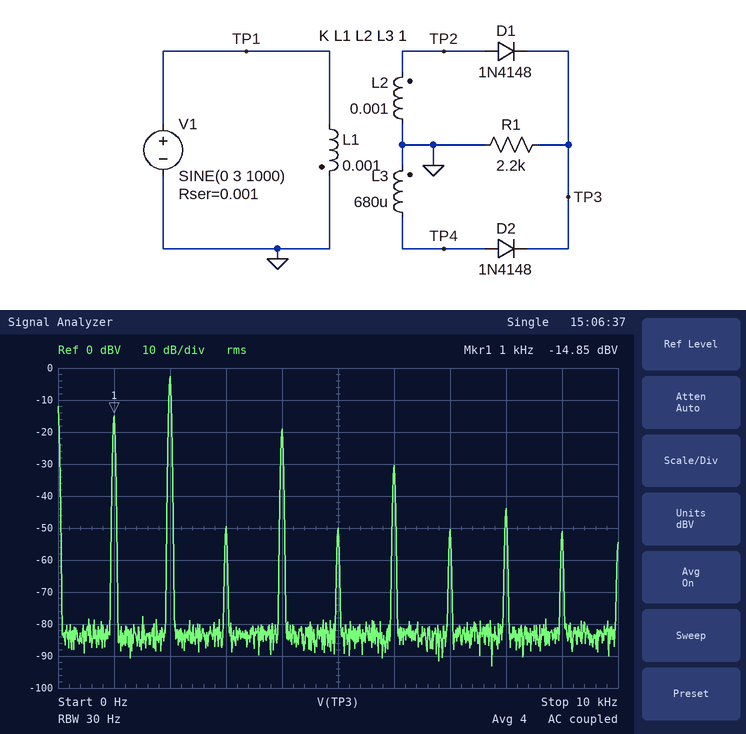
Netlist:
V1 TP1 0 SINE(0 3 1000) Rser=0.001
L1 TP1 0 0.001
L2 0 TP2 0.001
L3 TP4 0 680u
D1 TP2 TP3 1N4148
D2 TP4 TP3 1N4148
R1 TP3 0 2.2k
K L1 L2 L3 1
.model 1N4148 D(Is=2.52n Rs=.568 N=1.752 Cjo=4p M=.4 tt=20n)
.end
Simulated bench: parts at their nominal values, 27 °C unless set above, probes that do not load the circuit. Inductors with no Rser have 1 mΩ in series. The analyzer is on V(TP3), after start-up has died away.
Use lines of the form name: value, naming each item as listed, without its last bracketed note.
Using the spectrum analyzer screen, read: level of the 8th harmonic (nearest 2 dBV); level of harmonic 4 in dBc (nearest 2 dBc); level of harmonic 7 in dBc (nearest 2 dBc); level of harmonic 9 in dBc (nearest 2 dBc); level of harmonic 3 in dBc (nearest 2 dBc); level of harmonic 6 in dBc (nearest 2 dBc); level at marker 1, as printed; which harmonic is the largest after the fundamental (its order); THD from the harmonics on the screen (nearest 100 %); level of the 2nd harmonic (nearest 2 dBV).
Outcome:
level of the 8th harmonic: -44 dBV
level of harmonic 4 in dBc: -4 dBc
level of harmonic 7 in dBc: -36 dBc
level of harmonic 9 in dBc: -36 dBc
level of harmonic 3 in dBc: -34 dBc
level of harmonic 6 in dBc: -16 dBc
level at marker 1, as printed: -14.85 dBV
which harmonic is the largest after the fundamental: 2
THD from the harmonics on the screen: 400 %
level of the 2nd harmonic: -2 dBV
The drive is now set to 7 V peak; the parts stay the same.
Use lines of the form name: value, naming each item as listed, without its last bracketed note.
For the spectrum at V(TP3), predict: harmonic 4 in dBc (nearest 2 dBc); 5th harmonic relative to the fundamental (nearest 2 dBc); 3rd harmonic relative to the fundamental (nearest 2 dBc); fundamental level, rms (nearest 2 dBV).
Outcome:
harmonic 4 in dBc: -2 dBc
5th harmonic relative to the fundamental: -50 dBc
3rd harmonic relative to the fundamental: -48 dBc
fundamental level, rms: -8 dBV
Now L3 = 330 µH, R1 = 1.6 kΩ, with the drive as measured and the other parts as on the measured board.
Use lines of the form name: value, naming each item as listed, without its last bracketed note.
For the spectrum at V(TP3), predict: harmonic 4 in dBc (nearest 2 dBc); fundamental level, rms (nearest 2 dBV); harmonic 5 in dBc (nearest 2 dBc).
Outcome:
harmonic 4 in dBc: -14 dBc
fundamental level, rms: -8 dBV
harmonic 5 in dBc: -32 dBc
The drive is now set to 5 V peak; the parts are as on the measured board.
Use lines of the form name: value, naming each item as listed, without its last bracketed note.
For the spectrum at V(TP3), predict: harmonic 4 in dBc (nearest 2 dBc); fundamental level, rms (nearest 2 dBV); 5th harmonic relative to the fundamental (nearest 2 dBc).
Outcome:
harmonic 4 in dBc: -2 dBc
fundamental level, rms: -10 dBV
5th harmonic relative to the fundamental: -44 dBc
